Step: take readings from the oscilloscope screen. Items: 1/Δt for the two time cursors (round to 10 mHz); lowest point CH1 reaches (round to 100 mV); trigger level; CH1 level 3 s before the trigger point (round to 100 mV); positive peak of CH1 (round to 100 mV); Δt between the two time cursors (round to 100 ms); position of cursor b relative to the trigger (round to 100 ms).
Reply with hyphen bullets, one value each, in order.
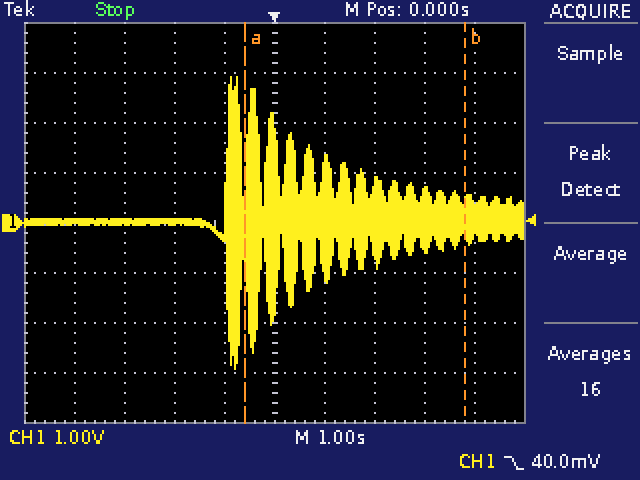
- 230 mHz
- -2.9 V
- 40.0 mV
- 0.0 V
- 2.9 V
- 4.4 s
- +3.8 s
